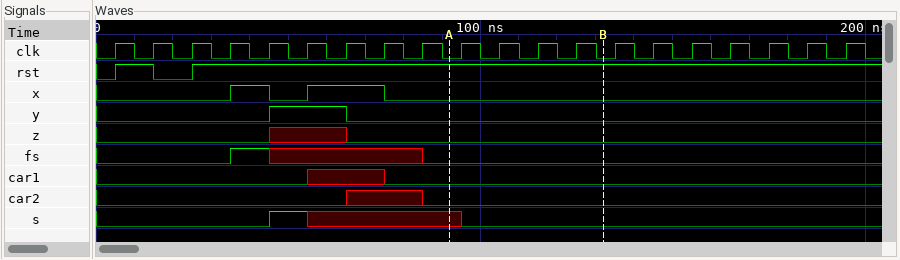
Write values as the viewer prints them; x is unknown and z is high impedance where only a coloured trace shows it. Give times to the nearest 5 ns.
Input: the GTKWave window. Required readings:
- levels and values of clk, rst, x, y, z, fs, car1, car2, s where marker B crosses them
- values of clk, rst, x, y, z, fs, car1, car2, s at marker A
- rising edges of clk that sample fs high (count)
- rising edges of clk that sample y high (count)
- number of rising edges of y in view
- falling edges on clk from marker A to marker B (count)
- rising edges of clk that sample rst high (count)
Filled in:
clk=0, rst=1, x=0, y=0, z=0, fs=0, car1=0, car2=0, s=0
clk=0, rst=1, x=0, y=0, z=0, fs=0, car1=0, car2=0, s=x
1
2
1
4
18
